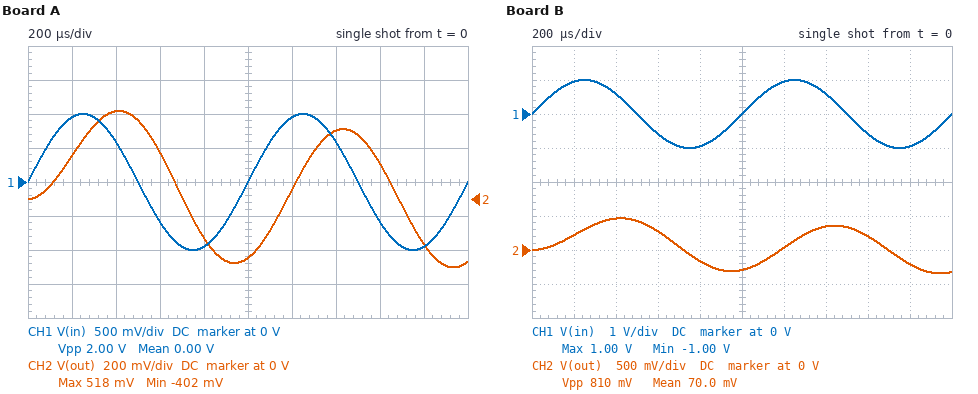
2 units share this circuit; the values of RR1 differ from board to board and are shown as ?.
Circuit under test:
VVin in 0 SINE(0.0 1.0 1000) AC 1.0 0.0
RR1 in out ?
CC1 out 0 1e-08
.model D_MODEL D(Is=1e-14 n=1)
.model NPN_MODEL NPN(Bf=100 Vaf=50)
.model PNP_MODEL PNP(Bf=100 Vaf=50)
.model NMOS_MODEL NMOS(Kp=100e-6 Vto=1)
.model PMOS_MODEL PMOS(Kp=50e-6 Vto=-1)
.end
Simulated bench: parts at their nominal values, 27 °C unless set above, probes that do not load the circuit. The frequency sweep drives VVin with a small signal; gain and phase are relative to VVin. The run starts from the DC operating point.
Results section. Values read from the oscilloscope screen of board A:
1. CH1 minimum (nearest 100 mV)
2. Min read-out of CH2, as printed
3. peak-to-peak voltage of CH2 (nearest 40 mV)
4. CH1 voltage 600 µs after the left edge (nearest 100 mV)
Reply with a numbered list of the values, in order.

1. -1.0 V
2. -402 mV
3. 920 mV
4. -600 mV
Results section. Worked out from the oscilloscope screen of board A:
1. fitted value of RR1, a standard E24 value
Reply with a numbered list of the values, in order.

1. 36 kΩ
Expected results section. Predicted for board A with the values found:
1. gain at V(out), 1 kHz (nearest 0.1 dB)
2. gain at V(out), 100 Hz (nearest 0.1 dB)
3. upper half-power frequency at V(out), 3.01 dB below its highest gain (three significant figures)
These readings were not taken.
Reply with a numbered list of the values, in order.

1. -7.9 dB
2. -0.2 dB
3. 442 Hz
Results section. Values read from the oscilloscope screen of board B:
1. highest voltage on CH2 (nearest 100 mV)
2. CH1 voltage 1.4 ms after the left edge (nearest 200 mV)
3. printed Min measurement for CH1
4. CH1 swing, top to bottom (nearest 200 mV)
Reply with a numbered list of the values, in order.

1. 500 mV
2. 600 mV
3. -1.00 V
4. 2.0 V
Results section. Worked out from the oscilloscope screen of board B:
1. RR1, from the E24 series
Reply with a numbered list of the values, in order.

1. 43 kΩ
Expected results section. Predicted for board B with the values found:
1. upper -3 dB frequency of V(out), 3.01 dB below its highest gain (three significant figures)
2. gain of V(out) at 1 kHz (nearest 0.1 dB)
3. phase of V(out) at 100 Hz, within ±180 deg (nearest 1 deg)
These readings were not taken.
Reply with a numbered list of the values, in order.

1. 370 Hz
2. -9.2 dB
3. -15 deg
